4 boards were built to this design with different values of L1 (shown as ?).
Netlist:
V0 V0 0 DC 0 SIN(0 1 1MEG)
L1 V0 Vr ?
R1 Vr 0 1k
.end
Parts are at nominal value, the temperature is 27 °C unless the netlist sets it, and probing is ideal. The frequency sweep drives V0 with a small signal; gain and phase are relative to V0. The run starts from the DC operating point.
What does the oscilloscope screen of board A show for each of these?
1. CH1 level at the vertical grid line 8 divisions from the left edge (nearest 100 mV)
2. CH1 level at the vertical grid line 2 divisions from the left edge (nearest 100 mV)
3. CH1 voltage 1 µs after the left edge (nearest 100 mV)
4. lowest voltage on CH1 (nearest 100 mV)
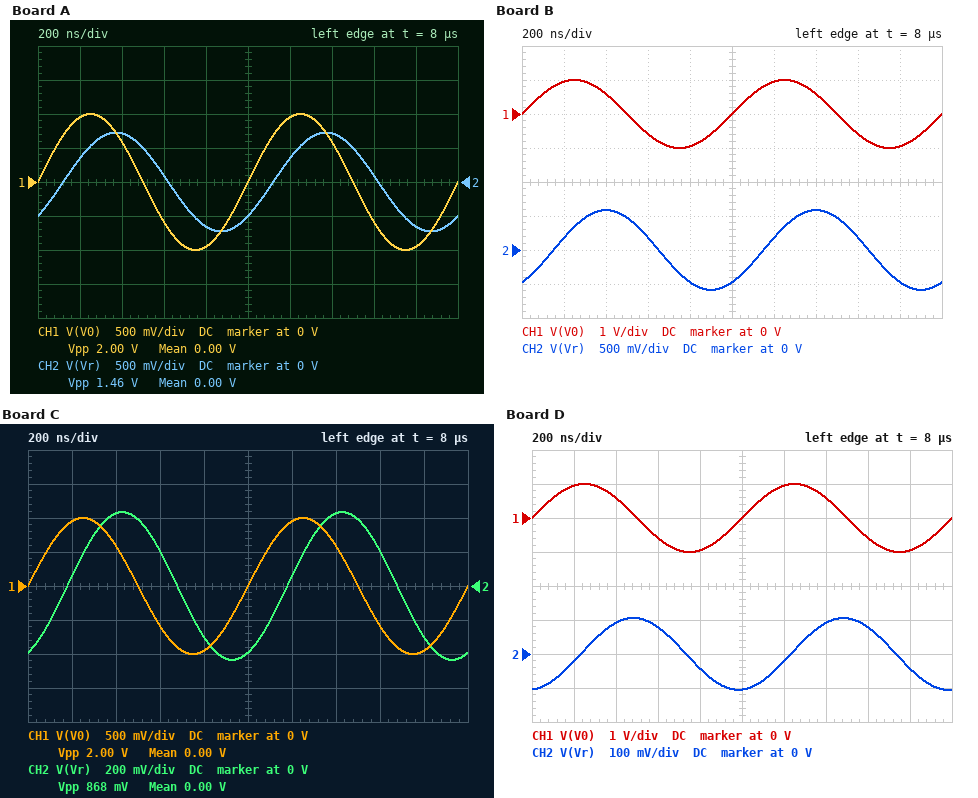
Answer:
-600 mV
600 mV
0 V
-1.0 V
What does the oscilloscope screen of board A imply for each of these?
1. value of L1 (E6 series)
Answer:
150 µH
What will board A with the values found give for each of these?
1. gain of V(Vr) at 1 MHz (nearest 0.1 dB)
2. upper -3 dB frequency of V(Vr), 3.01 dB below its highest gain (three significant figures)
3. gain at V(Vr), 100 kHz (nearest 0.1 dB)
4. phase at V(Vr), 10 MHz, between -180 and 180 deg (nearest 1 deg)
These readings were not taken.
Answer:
-2.8 dB
1.06 MHz
0 dB
-84 deg
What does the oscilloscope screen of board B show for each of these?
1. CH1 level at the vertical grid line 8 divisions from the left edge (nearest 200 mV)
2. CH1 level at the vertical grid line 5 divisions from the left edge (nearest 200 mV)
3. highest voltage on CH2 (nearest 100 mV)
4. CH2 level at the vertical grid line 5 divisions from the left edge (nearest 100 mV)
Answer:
-600 mV
0 V
600 mV
-500 mV
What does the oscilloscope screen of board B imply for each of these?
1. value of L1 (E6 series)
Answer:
220 µH
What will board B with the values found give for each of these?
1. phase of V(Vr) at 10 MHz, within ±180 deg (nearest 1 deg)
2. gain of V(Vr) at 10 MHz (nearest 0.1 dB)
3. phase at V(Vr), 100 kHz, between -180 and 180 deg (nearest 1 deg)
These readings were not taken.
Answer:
-86 deg
-22.8 dB
-8 deg
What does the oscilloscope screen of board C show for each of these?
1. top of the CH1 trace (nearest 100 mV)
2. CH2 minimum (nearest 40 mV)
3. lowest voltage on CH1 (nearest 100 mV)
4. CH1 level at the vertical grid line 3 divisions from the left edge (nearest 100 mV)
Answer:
1.0 V
-440 mV
-1.0 V
-600 mV
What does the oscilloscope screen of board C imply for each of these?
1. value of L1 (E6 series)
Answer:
330 µH
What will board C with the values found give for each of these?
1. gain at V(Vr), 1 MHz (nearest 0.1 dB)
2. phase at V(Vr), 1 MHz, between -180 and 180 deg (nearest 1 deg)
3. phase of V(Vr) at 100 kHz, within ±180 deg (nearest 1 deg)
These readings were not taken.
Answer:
-7.2 dB
-64 deg
-12 deg
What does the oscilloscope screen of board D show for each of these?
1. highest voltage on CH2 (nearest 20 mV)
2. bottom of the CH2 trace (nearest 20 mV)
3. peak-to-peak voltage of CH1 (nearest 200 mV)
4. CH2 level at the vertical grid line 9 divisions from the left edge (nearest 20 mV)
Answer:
100 mV
-100 mV
2.0 V
-40 mV
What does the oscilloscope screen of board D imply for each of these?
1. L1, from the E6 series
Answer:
1.5 mH
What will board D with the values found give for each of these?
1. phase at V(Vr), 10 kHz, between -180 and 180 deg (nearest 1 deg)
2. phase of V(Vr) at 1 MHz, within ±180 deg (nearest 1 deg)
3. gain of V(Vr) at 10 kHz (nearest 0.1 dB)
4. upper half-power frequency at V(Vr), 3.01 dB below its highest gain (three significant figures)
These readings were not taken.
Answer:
-5 deg
-84 deg
0 dB
106 kHz
